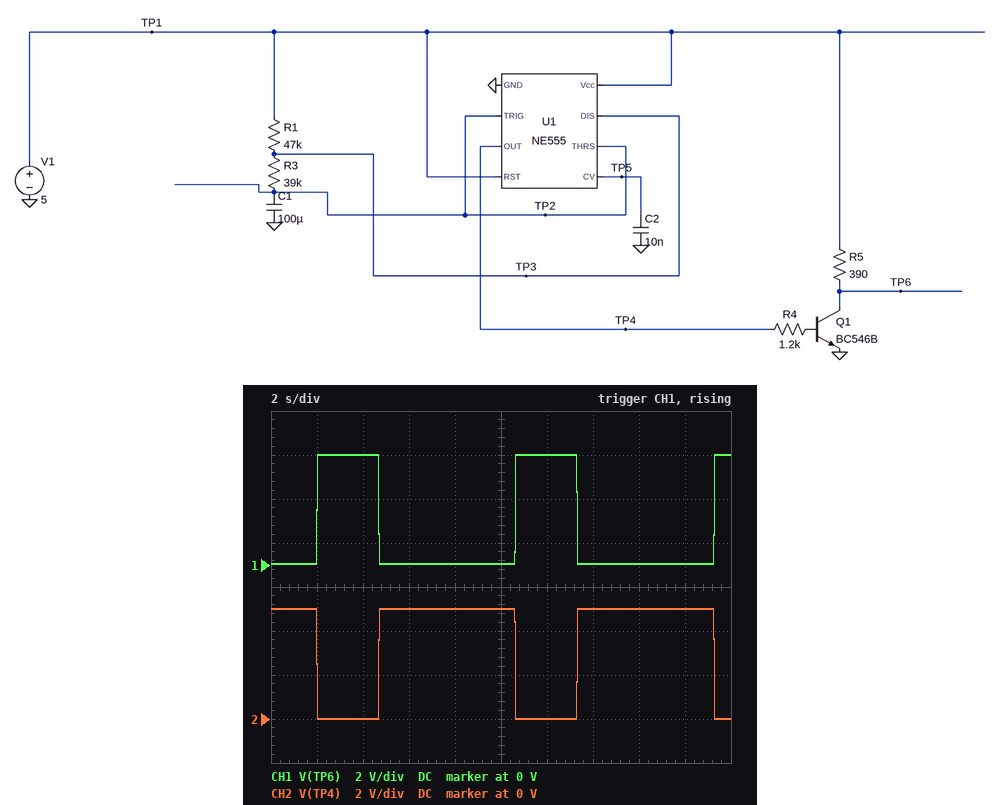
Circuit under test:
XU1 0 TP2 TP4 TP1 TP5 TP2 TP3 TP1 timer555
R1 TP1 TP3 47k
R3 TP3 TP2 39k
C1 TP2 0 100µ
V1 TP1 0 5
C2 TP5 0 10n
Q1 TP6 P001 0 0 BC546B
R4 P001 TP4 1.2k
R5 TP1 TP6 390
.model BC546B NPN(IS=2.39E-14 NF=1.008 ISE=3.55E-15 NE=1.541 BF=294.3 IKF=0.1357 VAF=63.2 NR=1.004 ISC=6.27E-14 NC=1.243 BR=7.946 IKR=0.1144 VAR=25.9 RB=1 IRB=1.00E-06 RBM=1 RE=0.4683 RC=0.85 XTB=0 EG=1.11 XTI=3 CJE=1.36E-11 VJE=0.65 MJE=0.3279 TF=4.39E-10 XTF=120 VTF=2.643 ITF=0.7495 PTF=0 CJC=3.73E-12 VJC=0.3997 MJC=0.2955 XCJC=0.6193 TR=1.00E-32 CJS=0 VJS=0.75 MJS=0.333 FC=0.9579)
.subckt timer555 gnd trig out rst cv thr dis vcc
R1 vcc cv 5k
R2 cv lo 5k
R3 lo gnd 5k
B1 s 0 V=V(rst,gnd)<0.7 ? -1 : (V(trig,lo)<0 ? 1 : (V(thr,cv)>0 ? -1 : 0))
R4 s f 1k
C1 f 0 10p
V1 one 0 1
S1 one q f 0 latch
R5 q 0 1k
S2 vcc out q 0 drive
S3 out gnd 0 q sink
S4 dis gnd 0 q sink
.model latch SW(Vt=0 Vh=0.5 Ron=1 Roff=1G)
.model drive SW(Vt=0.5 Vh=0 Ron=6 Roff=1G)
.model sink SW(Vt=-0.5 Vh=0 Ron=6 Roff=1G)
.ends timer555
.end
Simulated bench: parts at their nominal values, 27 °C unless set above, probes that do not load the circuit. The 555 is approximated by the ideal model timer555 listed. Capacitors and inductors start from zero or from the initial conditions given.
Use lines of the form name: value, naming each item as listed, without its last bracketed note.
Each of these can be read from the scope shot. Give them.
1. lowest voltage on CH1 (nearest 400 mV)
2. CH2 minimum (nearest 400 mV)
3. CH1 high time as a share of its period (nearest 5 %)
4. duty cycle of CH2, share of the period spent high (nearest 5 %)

lowest voltage on CH1: 0 V
CH2 minimum: 0 V
CH1 high time as a share of its period: 30 %
duty cycle of CH2, share of the period spent high: 70 %
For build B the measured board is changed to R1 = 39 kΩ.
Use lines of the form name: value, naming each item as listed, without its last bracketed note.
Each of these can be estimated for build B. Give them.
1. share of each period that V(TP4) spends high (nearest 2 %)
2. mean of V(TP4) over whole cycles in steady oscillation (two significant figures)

share of each period that V(TP4) spends high: 66 %
mean of V(TP4) over whole cycles in steady oscillation: 3.3 V
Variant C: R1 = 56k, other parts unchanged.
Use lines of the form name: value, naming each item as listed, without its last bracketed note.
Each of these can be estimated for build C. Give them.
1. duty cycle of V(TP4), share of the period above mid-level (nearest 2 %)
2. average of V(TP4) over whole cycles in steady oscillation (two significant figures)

duty cycle of V(TP4), share of the period above mid-level: 70 %
average of V(TP4) over whole cycles in steady oscillation: 3.5 V
